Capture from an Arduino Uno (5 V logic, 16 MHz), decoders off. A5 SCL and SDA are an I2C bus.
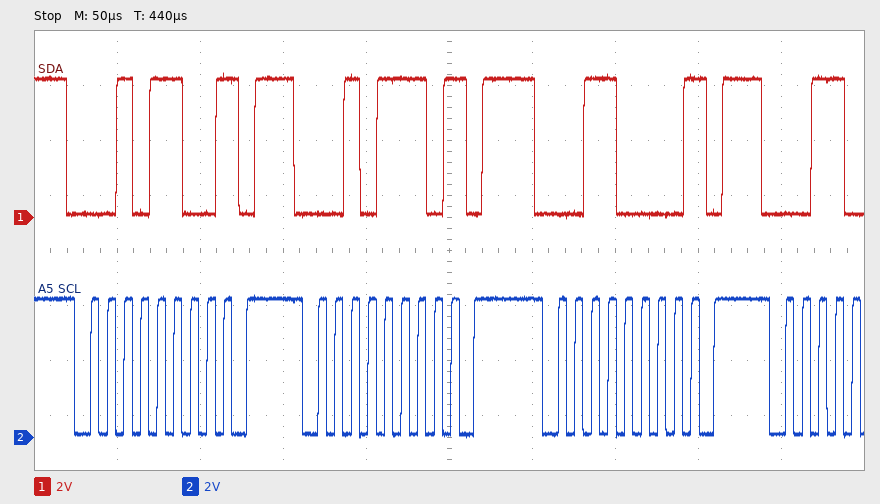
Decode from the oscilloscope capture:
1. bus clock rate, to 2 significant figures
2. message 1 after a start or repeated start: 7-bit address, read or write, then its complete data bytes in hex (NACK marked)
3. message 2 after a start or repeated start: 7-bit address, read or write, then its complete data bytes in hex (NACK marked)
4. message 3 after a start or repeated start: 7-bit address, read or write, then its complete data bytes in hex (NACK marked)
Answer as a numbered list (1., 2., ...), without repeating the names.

1. 100 kHz
2. 0x16 write NACK
3. 0x17 write NACK
4. 0x18 write NACK
